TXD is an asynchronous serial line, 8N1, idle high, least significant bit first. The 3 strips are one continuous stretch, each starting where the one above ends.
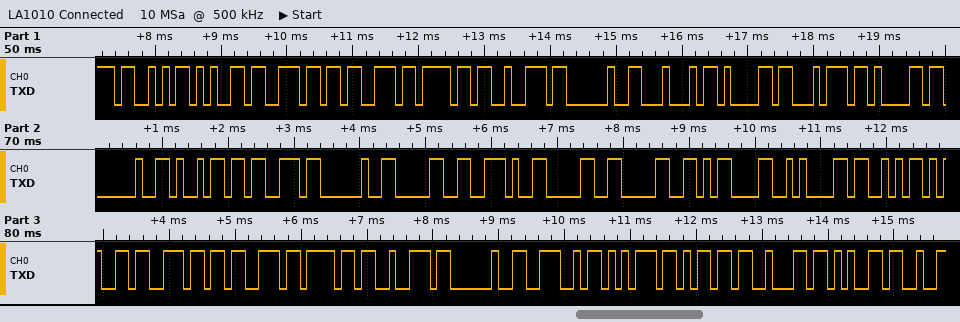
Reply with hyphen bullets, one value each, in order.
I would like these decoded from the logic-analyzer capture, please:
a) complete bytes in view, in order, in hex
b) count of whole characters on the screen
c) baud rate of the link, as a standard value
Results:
- 53 65 6E 73 6F 72 20 44 61 74 61 20 69 73 20 30 2E 30 30 0D 0A 53 65 6E 73 6F 72 20 4E 75 6D 62 65
- 33
- 9600 baud
